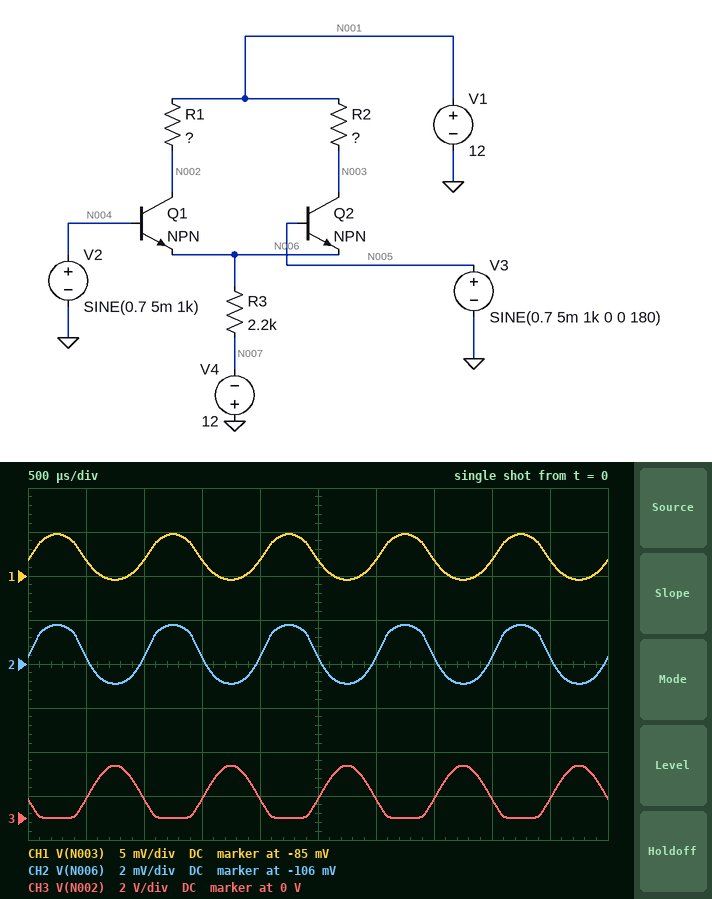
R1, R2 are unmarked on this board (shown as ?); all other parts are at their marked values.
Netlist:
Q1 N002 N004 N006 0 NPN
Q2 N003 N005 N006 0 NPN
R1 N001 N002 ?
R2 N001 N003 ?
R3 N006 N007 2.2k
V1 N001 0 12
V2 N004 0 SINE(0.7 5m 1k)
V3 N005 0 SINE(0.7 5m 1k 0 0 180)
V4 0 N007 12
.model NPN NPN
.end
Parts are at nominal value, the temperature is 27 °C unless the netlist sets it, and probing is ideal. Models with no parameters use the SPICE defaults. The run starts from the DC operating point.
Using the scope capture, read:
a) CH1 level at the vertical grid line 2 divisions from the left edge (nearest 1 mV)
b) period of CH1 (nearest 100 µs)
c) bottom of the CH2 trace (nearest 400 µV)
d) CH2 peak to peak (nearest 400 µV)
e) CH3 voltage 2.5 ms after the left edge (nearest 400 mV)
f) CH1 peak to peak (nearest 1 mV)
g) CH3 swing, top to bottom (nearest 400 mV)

-83 mV
1.0 ms
-106.8 mV
2.8 mV
800 mV
5 mV
2.4 V
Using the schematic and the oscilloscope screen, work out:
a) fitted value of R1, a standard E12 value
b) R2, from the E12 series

3.3 kΩ
22 kΩ
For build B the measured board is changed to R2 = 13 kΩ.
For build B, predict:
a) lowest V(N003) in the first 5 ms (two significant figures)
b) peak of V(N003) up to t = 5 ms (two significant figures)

-81 mV
-73 mV
